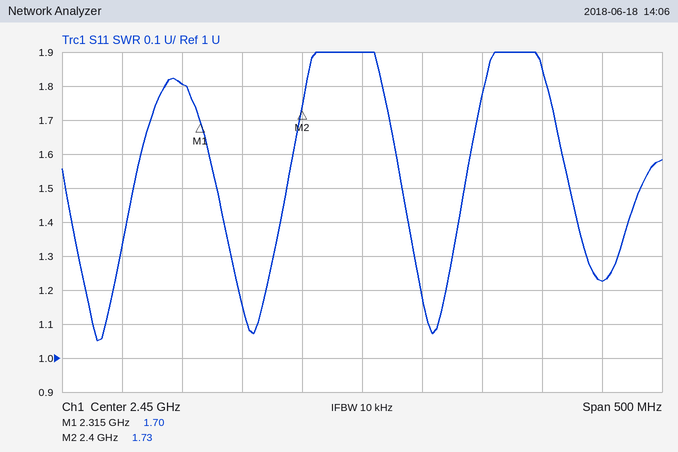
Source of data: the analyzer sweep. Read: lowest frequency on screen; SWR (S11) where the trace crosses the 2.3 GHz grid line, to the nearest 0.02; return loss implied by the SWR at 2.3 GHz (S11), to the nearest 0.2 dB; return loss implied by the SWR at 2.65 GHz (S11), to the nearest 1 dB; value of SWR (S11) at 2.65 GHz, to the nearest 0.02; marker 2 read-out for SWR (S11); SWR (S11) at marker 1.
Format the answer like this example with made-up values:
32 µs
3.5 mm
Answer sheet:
2.2 GHz
1.80
10.8 dB
20 dB
1.22
1.73
1.70
